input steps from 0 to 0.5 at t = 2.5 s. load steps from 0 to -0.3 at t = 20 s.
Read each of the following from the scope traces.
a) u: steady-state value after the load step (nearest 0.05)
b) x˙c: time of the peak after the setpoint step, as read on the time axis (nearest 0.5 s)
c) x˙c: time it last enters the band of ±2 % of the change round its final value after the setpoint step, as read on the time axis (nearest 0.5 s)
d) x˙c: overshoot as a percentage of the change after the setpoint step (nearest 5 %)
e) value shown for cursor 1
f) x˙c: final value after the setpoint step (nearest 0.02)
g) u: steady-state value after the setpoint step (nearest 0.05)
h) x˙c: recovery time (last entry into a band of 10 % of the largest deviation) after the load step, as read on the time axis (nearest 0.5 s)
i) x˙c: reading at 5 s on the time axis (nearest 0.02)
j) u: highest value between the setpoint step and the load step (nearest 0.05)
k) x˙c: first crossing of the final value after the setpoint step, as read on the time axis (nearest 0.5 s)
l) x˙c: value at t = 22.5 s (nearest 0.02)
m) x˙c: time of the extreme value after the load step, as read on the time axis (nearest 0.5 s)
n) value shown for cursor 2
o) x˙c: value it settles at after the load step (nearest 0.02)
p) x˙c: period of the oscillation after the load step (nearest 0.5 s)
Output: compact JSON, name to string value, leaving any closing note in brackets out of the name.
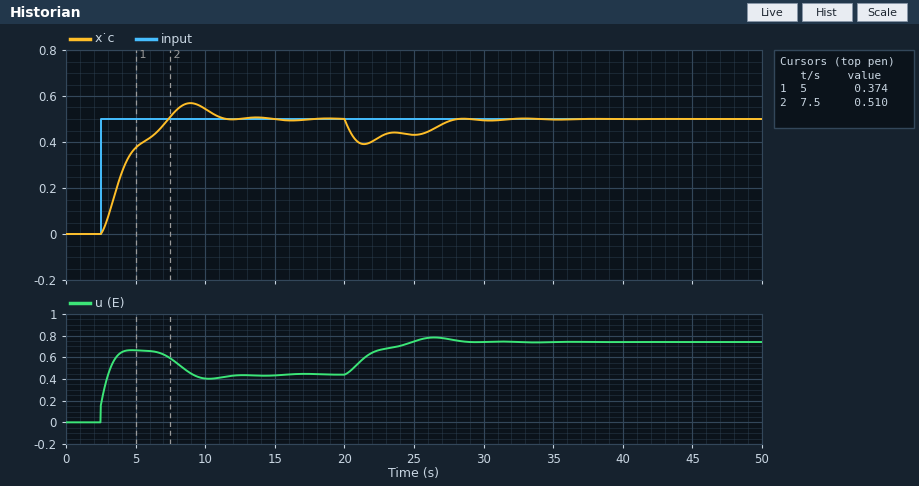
{"u: steady-state value after the load step": "0.75", "x˙c: time of the peak after the setpoint step, as read on the time axis": "9.0 s", "x˙c: time it last enters the band of ±2 % of the change round its final value after the setpoint step, as read on the time axis": "11.0 s", "x˙c: overshoot as a percentage of the change after the setpoint step": "15 %", "value shown for cursor 1": "0.374", "x˙c: final value after the setpoint step": "0.50", "u: steady-state value after the setpoint step": "0.45", "x˙c: recovery time (last entry into a band of 10 % of the largest deviation) after the load step, as read on the time axis": "27.5 s", "x˙c: reading at 5 s on the time axis": "0.38", "u: highest value between the setpoint step and the load step": "0.65", "x˙c: first crossing of the final value after the setpoint step, as read on the time axis": "7.5 s", "x˙c: value at t = 22.5 s": "0.42", "x˙c: time of the extreme value after the load step, as read on the time axis": "21.5 s", "value shown for cursor 2": "0.510", "x˙c: value it settles at after the load step": "0.50", "x˙c: period of the oscillation after the load step": "3.5 s"}
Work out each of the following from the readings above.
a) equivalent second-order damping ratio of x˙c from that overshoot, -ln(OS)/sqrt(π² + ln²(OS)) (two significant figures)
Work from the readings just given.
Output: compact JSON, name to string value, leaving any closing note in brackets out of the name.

{"equivalent second-order damping ratio of x˙c from that overshoot, -ln(OS)/sqrt(π² + ln²(OS))": "0.52"}
